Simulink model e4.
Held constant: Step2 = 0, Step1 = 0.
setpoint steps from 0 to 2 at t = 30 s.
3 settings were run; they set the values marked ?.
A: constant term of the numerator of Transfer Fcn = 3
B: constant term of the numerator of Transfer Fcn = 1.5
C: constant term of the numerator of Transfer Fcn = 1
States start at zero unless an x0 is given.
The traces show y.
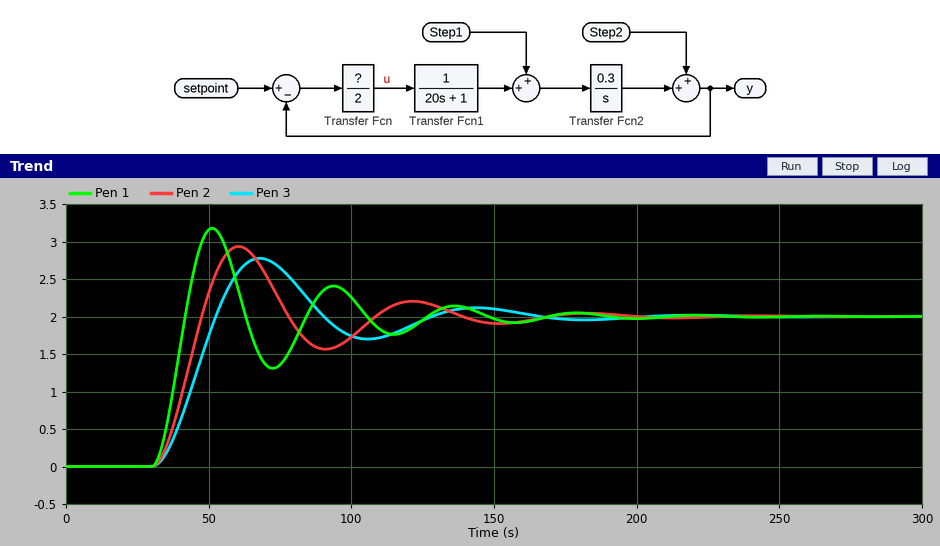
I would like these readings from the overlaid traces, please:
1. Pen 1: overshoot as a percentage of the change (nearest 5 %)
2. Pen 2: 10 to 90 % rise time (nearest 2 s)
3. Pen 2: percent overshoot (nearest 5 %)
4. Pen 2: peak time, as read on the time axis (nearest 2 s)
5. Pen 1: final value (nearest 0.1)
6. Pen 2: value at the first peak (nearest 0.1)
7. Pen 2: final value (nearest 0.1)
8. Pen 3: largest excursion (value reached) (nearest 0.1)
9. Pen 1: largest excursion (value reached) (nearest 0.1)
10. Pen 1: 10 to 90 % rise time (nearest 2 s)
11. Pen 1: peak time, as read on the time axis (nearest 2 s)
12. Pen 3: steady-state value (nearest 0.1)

60 %
12 s
45 %
60 s
2.0
2.9
2.0
2.8
3.2
8 s
52 s
2.0
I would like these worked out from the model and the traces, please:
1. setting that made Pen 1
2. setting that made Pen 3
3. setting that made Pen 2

A
C
B
